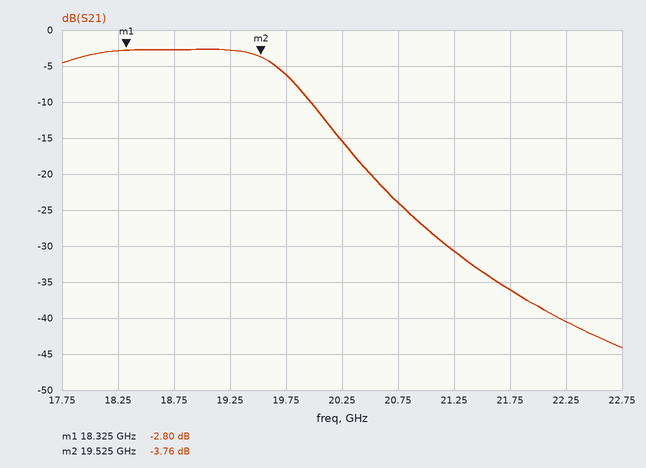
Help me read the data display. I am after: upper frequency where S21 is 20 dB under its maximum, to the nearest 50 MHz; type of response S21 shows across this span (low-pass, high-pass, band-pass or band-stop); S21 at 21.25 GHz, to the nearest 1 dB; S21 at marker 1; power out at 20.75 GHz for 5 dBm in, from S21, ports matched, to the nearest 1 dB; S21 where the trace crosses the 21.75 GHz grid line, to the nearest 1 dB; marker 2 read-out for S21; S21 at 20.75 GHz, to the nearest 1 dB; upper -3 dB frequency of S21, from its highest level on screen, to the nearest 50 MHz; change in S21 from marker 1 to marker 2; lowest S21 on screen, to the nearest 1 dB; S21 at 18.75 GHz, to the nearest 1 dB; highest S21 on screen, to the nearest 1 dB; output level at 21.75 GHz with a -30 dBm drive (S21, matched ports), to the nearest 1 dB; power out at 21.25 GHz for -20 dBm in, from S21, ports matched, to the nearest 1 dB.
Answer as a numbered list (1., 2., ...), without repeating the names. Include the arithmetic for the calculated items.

1. 20.65 GHz
2. low-pass
3. -31 dB
4. -2.80 dB
5. 5 dBm + (-24 dB) = -19 dBm
6. -36 dB
7. -3.76 dB
8. -24 dB
9. 19.70 GHz
10. -3.76 − (-2.8) = -0.96 dB
11. -44 dB
12. -3 dB
13. -3 dB
14. -30 dBm + (-36 dB) = -66 dBm
15. -20 dBm + (-31 dB) = -51 dBm
